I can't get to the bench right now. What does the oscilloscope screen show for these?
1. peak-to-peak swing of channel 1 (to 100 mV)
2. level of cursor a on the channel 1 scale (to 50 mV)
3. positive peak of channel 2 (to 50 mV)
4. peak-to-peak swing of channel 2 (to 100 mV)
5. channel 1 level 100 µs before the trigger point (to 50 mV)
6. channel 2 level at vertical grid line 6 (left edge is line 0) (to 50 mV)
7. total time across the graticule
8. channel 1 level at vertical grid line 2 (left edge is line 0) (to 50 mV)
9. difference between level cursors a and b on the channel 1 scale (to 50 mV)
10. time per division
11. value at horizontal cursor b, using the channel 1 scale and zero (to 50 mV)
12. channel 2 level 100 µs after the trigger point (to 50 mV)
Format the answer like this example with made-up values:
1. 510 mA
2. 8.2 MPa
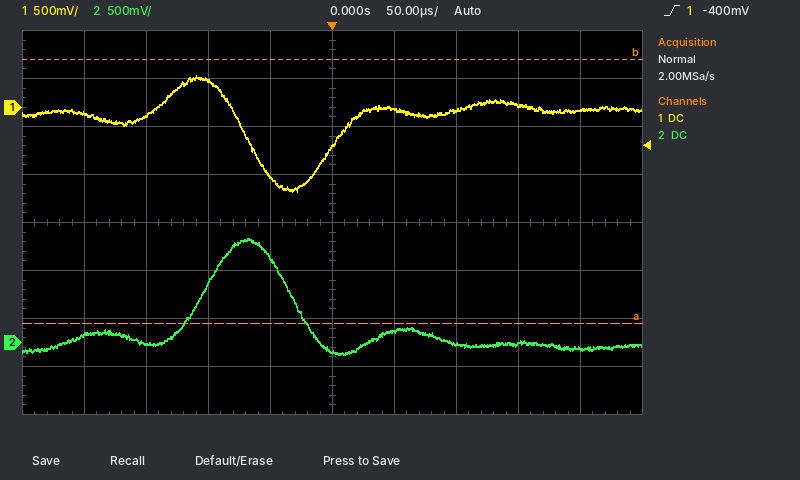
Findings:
1. 1.20 V
2. -2.25 V
3. 1.10 V
4. 1.20 V
5. 300 mV
6. 100 mV
7. 500 µs
8. -100 mV
9. 2.75 V
10. 50 µs
11. 500 mV
12. 0 mV
